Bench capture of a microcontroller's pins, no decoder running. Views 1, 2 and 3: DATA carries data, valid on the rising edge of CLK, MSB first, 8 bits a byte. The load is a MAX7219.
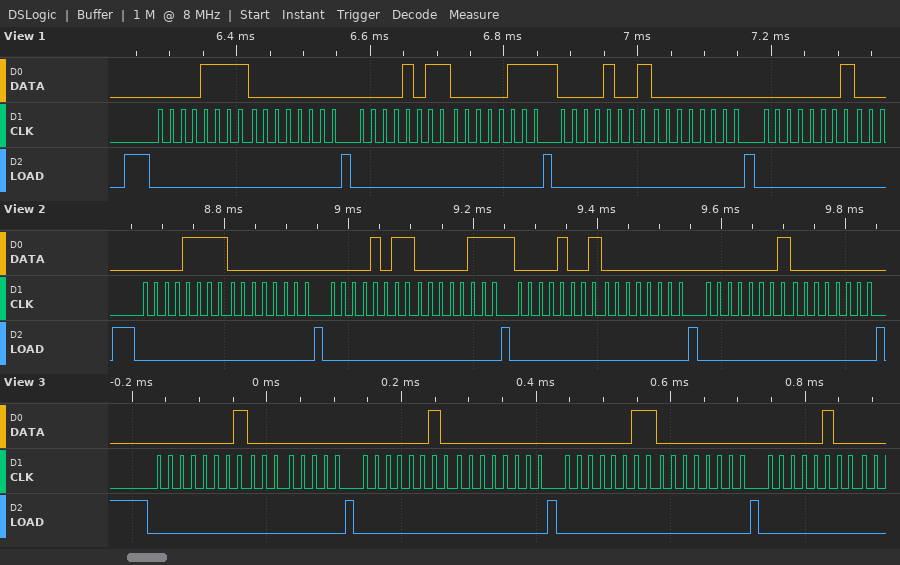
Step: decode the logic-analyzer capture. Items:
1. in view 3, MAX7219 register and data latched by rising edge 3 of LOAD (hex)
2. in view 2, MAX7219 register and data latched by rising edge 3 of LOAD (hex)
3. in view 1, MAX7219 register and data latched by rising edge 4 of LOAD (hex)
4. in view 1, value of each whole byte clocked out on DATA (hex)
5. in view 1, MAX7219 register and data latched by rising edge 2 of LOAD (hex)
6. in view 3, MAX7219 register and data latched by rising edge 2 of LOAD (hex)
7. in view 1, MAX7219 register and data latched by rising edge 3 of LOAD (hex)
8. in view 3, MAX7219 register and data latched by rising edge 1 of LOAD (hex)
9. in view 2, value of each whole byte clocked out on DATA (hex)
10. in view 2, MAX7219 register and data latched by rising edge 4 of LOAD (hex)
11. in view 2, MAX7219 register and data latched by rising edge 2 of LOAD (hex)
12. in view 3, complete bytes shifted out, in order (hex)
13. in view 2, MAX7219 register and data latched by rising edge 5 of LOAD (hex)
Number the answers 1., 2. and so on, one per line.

1. register 0x3, data 0x00
2. register 0xB, data 0x07
3. register 0x9, data 0x00
4. 0F 00 0B 07 09 00 01
5. register 0xF, data 0x00
6. register 0x2, data 0x00
7. register 0xB, data 0x07
8. register 0x1, data 0x00
9. 0F 00 0B 07 09 00 01 00
10. register 0x9, data 0x00
11. register 0xF, data 0x00
12. 0x01 0x00 0x02 0x00 0x03 0x00 0x04
13. register 0x1, data 0x00
